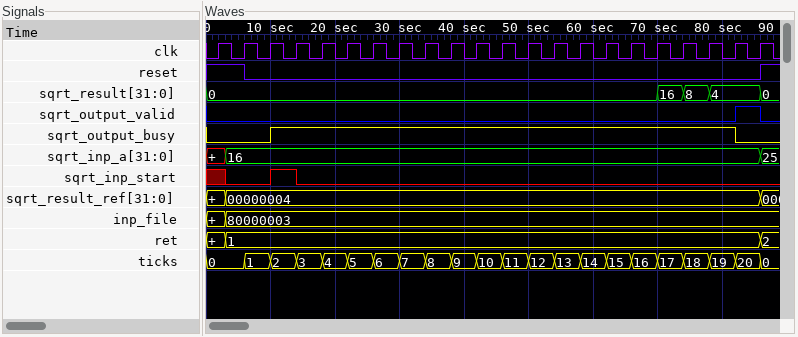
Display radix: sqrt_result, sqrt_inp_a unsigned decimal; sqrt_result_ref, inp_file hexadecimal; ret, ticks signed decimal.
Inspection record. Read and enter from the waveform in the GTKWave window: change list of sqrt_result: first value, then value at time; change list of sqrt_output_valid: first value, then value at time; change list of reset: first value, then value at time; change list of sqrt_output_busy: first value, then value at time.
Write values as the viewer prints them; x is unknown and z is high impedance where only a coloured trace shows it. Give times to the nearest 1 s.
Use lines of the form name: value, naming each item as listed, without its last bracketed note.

change list of sqrt_result: first value, then value at time: 0, 16 at 70 s, 8 at 74 s, 4 at 78 s, 0 at 86 s
change list of sqrt_output_valid: first value, then value at time: 0, 1 at 82 s, 0 at 86 s
change list of reset: first value, then value at time: 1, 0 at 6 s, 1 at 86 s
change list of sqrt_output_busy: first value, then value at time: 0, 1 at 10 s, 0 at 82 s
